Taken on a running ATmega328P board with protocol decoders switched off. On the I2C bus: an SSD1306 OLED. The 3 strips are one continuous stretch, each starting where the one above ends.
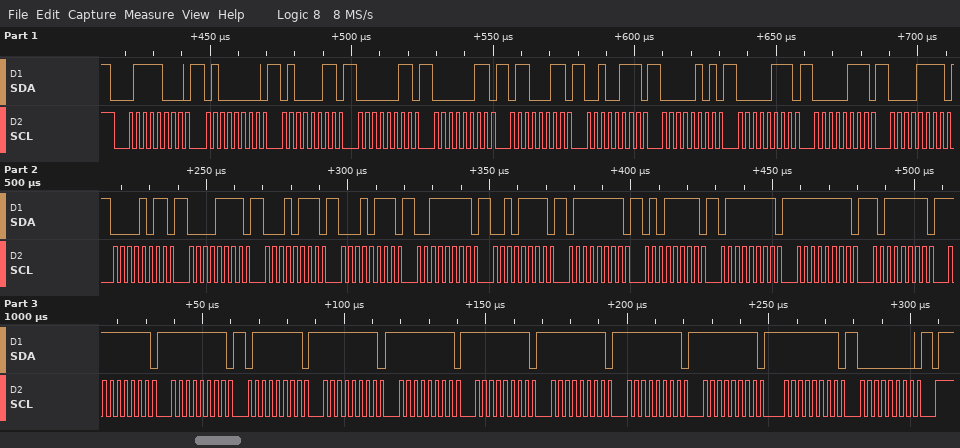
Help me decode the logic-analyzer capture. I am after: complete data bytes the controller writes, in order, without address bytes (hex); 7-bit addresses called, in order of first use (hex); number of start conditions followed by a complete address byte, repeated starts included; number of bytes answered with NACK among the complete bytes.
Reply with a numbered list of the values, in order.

1. 40 43 03 03 63 27 05 07 07 0F 0B 0F 17 17 3F 2F 7F 5F 7F FF BF FF FF 7F FF FF FF FF FF FF FF 00
2. 0x3C
3. 1
4. 0
